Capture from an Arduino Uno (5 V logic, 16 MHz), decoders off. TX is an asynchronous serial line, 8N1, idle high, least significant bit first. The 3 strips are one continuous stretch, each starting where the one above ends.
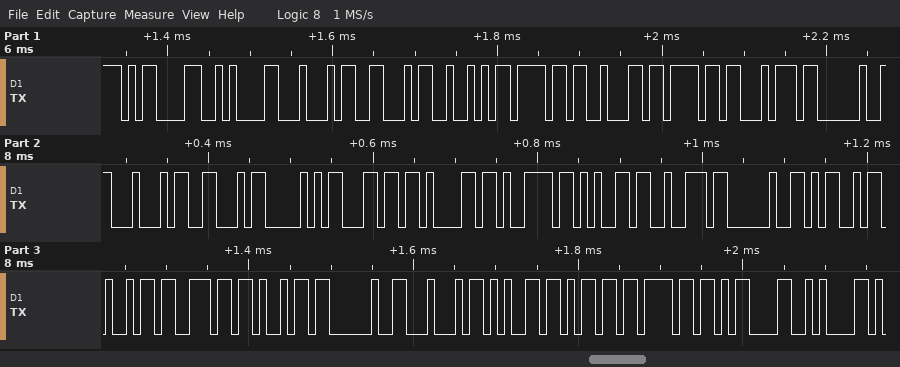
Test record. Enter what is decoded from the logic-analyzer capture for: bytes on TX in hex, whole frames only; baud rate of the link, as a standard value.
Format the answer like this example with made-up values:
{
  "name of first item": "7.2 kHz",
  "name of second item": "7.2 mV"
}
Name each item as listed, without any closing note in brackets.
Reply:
{
  "bytes on TX in hex, whole frames only": "0D 0A 44 46 52 6F 62 6F 74 20 44 46 50 6C 61 79 65 72 20 4D 69 6E 69 20 44 65 6D 6F 0D 0A",
  "baud rate of the link, as a standard value": "115200 baud"
}
